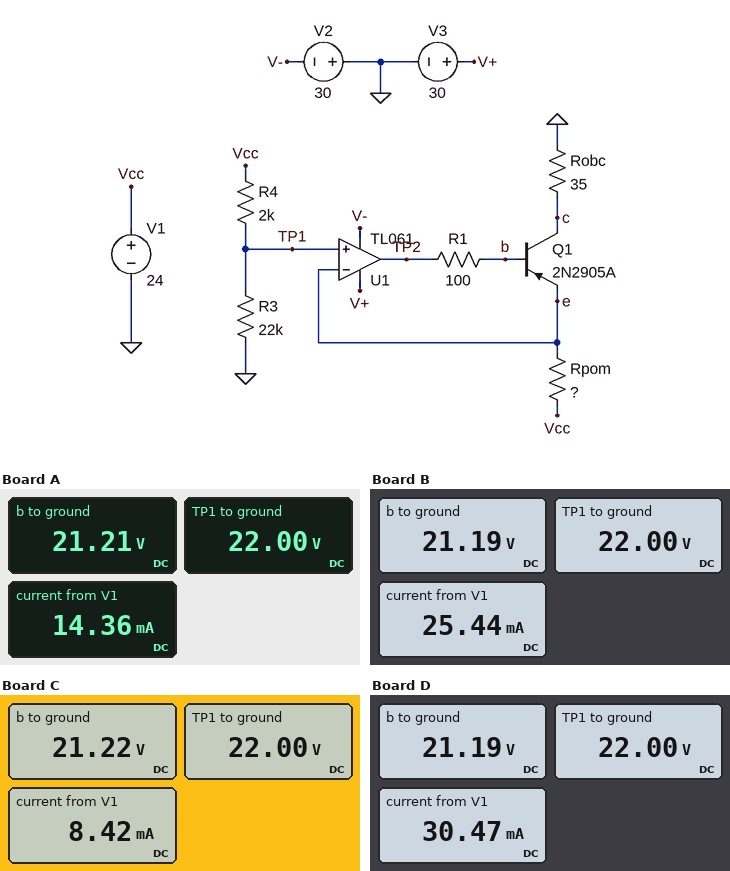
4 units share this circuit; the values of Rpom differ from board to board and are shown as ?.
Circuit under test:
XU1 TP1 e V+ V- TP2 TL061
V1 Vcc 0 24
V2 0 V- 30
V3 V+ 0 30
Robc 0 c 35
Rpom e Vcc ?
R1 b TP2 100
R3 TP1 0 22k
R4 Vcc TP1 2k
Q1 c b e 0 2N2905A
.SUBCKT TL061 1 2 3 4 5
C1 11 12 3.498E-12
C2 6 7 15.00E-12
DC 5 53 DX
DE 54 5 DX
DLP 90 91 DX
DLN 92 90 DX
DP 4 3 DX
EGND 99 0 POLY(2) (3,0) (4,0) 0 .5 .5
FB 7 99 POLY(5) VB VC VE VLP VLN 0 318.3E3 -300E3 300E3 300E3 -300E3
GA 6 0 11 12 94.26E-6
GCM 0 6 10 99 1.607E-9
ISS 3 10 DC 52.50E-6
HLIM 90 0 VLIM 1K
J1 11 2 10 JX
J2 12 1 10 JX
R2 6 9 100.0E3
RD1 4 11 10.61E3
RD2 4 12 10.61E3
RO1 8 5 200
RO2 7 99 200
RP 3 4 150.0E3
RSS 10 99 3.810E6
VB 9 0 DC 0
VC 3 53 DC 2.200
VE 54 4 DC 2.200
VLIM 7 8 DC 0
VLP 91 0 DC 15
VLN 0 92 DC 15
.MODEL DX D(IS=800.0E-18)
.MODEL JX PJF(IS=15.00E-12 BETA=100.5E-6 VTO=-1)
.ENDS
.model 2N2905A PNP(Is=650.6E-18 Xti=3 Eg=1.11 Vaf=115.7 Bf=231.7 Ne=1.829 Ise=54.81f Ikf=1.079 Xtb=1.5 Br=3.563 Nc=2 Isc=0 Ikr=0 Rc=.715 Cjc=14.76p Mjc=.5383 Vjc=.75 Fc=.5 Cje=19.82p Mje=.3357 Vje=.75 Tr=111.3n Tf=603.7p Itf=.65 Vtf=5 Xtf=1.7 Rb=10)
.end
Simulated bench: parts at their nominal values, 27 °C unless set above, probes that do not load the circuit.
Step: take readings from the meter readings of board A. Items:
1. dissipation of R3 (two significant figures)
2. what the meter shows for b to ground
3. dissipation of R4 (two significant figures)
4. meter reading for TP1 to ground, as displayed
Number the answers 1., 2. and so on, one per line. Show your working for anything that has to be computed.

1. (22 V)^2 / 22 kΩ = 22 mW
2. 21.21 V
3. (24 V - 22 V)^2 / 2 kΩ = 2.0 mW
4. 22.00 V
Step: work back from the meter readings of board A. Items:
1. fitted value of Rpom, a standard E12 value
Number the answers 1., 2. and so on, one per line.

1. 150 Ω
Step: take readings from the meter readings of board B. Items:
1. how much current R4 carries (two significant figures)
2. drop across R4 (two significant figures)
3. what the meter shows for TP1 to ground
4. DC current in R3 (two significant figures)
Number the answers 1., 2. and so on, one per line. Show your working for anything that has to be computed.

1. (24 V - 22 V) / 2 kΩ = 1.0 mA
2. 24 V - 22 V = 2.0 V
3. 22.00 V
4. (22 V) / 22 kΩ = 1.0 mA
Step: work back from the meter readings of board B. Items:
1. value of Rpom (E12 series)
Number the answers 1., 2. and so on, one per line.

1. 82 Ω
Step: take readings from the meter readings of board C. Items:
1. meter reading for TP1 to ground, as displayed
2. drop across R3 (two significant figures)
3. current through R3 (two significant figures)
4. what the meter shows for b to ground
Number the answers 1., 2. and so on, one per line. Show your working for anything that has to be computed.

1. 22.00 V
2. 22 V = 22 V
3. (22 V) / 22 kΩ = 1.0 mA
4. 21.22 V
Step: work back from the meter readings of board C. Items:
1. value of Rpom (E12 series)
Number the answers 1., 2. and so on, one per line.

1. 270 Ω
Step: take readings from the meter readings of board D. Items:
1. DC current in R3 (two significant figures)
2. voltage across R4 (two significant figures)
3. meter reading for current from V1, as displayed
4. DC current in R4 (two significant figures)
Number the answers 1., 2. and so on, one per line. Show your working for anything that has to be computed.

1. (22 V) / 22 kΩ = 1.0 mA
2. 24 V - 22 V = 2.0 V
3. 30.47 mA
4. (24 V - 22 V) / 2 kΩ = 1.0 mA
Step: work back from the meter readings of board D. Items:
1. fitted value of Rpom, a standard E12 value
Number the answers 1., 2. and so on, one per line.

1. 68 Ω
